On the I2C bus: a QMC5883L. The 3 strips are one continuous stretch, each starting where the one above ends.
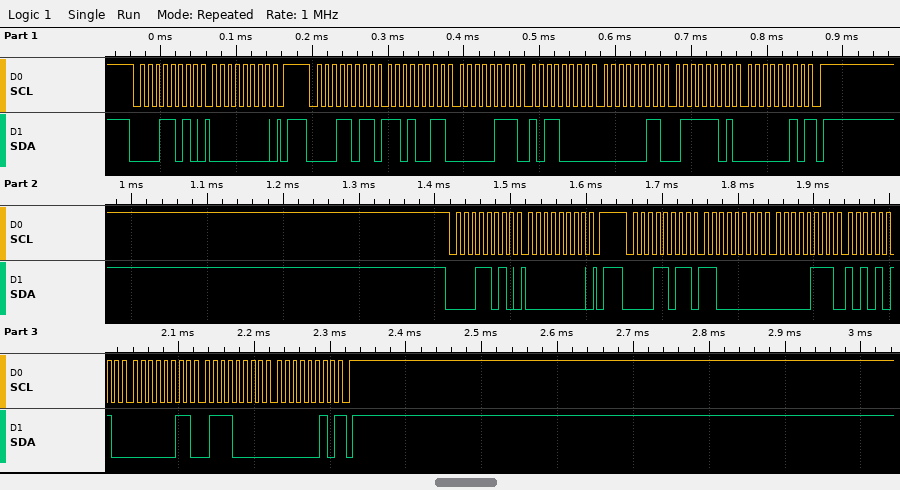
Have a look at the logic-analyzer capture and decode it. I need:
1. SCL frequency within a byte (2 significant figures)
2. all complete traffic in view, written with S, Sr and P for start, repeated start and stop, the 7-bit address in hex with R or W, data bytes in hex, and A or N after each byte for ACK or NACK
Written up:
100 kHz
S 0DW A 00 A P S 0DR A D3 A 07 A B0 A 03 A 7D A 02 N P S 0DW A 00 A P S 0DR A C0 A 07 A AA A 03 A 70 A 02 N P
